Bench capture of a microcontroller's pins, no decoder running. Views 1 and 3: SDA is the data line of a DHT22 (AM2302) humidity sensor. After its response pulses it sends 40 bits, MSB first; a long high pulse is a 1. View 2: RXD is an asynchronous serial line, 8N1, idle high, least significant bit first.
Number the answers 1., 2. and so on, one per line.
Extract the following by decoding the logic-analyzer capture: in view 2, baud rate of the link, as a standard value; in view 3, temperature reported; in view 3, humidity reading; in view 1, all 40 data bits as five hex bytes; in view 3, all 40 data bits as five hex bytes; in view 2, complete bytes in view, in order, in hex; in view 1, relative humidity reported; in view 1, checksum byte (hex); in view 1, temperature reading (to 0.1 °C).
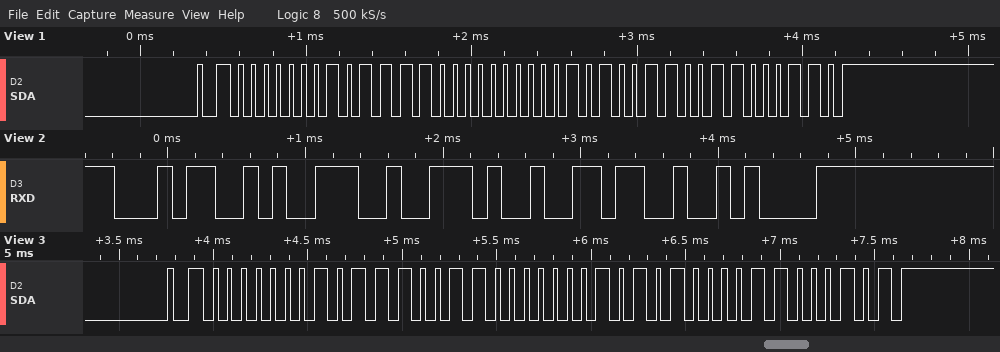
1. 9600 baud
2. 33.6 °C
3. 37.1 %
4. 01 78 01 4C C6
5. 01 73 01 50 C5
6. 34 39 2E 36 0A
7. 37.6 %
8. 0xC6
9. 33.2 °C
